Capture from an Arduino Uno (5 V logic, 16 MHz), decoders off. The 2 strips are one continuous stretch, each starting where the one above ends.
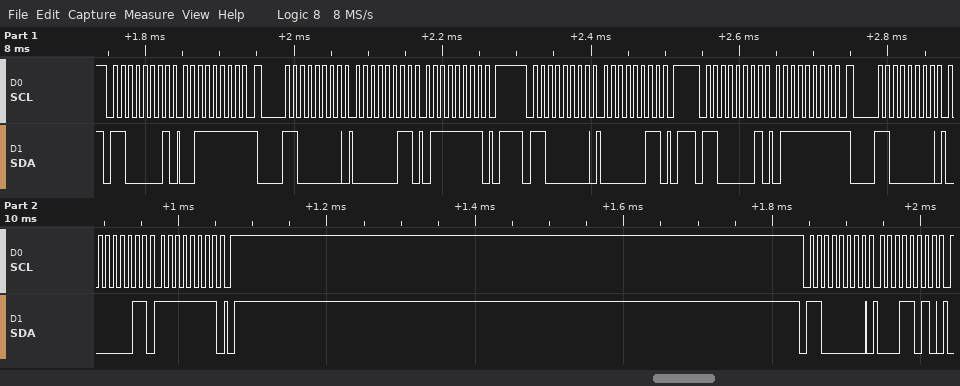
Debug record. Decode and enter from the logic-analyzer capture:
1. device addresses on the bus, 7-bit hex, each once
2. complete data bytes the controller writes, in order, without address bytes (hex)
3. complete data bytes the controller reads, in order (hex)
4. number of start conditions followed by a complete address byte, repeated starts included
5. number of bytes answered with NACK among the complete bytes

0x60
03 7F 03 03 FF 1A
3F 7F
6
2
